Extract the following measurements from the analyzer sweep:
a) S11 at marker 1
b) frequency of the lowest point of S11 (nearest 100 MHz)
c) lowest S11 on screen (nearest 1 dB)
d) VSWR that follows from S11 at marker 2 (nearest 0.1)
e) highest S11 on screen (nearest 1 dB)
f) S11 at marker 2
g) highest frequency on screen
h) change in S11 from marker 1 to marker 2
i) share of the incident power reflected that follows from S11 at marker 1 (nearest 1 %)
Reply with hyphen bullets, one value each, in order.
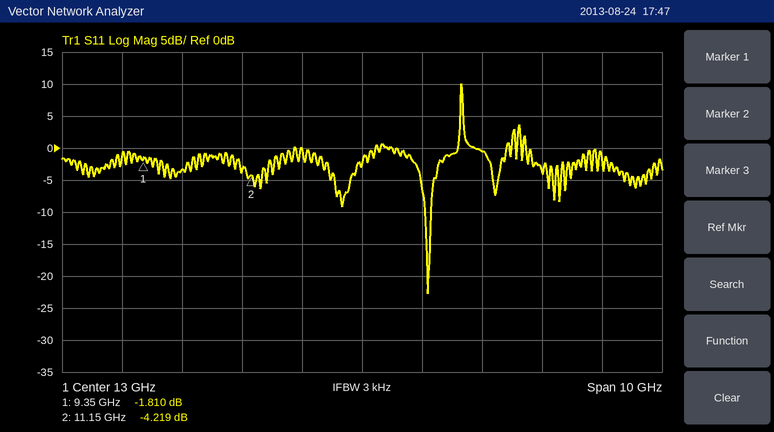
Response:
- -1.810 dB
- 14.1 GHz
- -23 dB
- 4.2
- 10 dB
- -4.219 dB
- 18 GHz
- -2.409 dB
- 66 %
